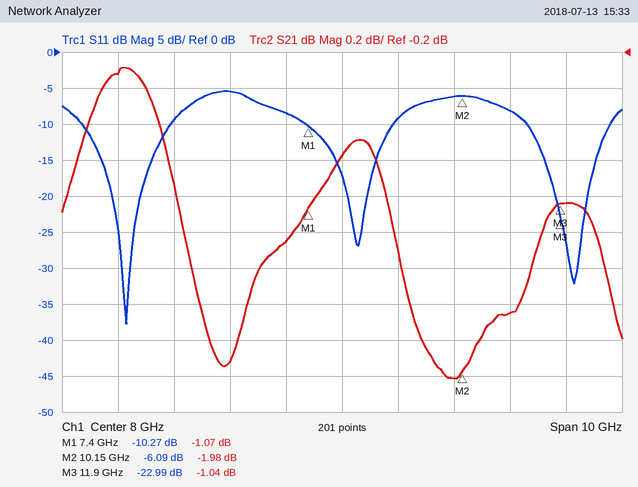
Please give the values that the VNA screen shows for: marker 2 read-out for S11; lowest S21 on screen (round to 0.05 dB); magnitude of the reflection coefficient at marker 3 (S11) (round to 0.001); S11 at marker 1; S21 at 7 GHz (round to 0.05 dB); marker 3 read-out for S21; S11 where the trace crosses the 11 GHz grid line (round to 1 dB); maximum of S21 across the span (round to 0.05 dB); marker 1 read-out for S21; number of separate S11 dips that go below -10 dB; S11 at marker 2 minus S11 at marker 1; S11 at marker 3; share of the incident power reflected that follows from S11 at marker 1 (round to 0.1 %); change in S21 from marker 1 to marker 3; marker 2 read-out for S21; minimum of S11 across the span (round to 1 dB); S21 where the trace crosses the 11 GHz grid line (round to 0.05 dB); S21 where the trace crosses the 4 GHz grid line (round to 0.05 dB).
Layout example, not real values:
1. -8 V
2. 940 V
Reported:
1. -6.09 dB
2. -2.00 dB
3. 0.071
4. -10.27 dB
5. -1.25 dB
6. -1.04 dB
7. -8 dB
8. -0.30 dB
9. -1.07 dB
10. 3
11. 4.18 dB
12. -22.99 dB
13. 9.4 %
14. 0.03 dB
15. -1.98 dB
16. -38 dB
17. -1.65 dB
18. -0.30 dB
